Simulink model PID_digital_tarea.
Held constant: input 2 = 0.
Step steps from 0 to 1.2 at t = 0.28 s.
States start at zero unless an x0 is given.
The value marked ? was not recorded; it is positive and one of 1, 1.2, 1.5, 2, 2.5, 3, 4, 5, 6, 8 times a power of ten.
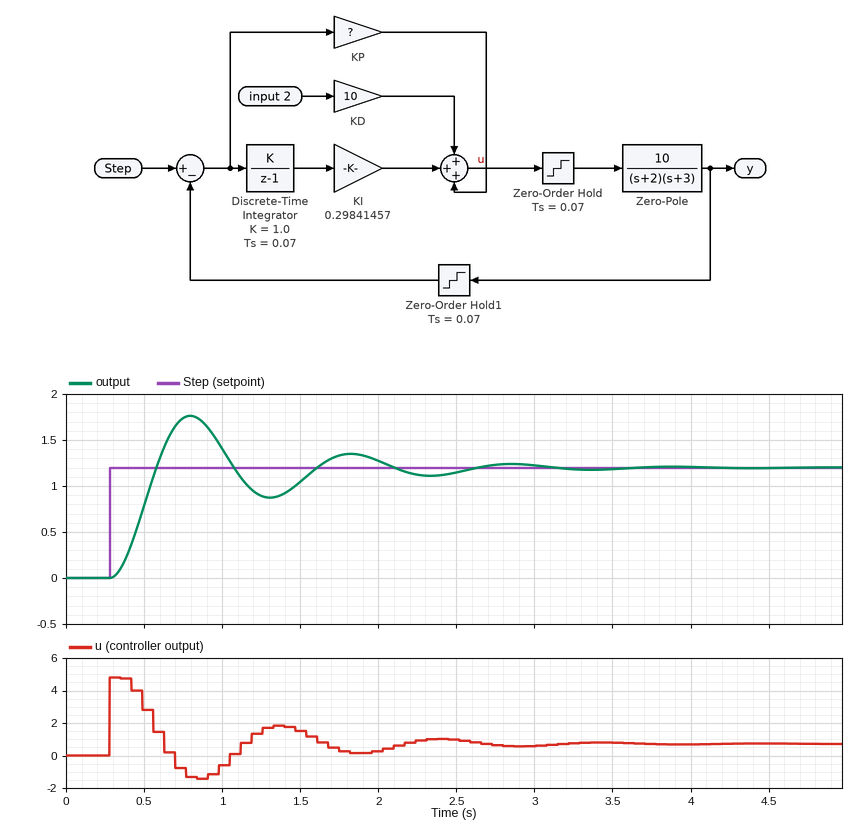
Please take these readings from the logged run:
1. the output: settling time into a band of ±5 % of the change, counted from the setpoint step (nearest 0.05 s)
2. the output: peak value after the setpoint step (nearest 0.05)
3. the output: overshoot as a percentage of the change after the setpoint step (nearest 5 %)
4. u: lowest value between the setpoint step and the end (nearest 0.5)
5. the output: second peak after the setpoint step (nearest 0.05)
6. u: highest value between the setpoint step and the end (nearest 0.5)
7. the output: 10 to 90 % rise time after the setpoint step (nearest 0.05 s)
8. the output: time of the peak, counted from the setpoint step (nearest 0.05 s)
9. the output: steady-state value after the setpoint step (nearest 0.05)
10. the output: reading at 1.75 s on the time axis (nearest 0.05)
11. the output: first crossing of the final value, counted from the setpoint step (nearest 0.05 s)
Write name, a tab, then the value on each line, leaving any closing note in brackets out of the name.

the output: settling time into a band of ±5 % of the change, counted from the setpoint step	2.20 s
the output: peak value after the setpoint step	1.75
the output: overshoot as a percentage of the change after the setpoint step	45 %
u: lowest value between the setpoint step and the end	-1.5
the output: second peak after the setpoint step	1.35
u: highest value between the setpoint step and the end	5.0
the output: 10 to 90 % rise time after the setpoint step	0.20 s
the output: time of the peak, counted from the setpoint step	0.50 s
the output: steady-state value after the setpoint step	1.20
the output: reading at 1.75 s on the time axis	1.35
the output: first crossing of the final value, counted from the setpoint step	0.30 s
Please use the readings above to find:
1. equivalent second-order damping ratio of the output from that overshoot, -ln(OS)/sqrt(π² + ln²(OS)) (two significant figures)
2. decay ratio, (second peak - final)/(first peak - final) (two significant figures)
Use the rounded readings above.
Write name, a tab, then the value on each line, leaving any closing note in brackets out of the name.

equivalent second-order damping ratio of the output from that overshoot, -ln(OS)/sqrt(π² + ln²(OS))	0.25
decay ratio, (second peak - final)/(first peak - final)	0.27
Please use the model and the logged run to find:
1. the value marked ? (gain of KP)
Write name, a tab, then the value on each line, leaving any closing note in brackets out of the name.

the value marked ?	4
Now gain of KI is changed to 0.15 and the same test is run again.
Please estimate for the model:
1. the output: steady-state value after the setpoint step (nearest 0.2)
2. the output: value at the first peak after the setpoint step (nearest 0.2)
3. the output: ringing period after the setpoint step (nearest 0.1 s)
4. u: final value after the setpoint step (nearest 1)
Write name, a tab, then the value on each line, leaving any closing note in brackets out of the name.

the output: steady-state value after the setpoint step	1.2
the output: value at the first peak after the setpoint step	1.6
the output: ringing period after the setpoint step	1.0 s
u: final value after the setpoint step	1
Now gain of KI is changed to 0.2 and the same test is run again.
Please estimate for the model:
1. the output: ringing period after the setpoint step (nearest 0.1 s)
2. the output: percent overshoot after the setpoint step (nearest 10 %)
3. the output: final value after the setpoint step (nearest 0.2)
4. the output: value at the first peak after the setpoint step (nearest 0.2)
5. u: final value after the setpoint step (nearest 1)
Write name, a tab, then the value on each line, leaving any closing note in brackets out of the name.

the output: ringing period after the setpoint step	1.0 s
the output: percent overshoot after the setpoint step	40 %
the output: final value after the setpoint step	1.2
the output: value at the first peak after the setpoint step	1.6
u: final value after the setpoint step	1
